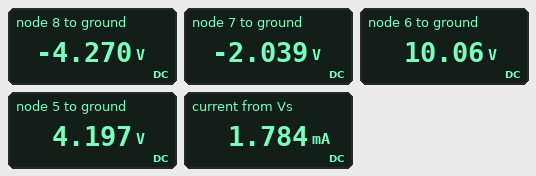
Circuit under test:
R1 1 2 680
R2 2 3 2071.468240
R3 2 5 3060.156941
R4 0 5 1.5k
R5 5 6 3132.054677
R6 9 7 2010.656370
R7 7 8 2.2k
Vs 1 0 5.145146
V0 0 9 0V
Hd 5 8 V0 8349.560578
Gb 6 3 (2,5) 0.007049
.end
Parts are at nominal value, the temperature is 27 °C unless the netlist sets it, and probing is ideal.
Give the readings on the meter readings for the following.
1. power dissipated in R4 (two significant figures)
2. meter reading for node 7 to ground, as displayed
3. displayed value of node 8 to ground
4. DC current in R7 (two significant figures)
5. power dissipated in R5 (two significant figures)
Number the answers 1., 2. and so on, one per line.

1. 12 mW
2. -2.039 V
3. -4.270 V
4. 1.0 mA
5. 11 mW
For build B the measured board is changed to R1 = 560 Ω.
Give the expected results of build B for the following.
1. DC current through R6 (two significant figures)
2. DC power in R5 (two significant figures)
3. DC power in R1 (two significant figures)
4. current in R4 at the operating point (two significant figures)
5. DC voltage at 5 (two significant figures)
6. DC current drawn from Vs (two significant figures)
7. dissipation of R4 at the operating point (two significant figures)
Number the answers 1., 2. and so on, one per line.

1. 1.1 mA
2. 12 mW
3. 1.9 mW
4. 2.9 mA
5. 4.4 V
6. 1.9 mA
7. 13 mW
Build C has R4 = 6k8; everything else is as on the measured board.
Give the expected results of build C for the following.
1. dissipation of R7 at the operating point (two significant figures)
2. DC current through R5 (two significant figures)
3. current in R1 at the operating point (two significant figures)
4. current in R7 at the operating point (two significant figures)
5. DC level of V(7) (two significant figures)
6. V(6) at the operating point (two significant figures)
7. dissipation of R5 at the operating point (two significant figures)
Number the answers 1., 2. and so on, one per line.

1. 3.8 mW
2. 540 µA
3. 510 µA
4. 1.3 mA
5. -2.6 V
6. 3.7 V
7. 900 µW
